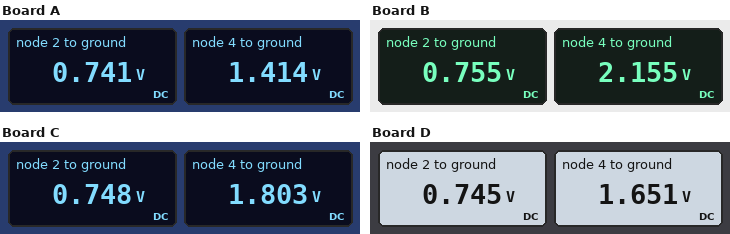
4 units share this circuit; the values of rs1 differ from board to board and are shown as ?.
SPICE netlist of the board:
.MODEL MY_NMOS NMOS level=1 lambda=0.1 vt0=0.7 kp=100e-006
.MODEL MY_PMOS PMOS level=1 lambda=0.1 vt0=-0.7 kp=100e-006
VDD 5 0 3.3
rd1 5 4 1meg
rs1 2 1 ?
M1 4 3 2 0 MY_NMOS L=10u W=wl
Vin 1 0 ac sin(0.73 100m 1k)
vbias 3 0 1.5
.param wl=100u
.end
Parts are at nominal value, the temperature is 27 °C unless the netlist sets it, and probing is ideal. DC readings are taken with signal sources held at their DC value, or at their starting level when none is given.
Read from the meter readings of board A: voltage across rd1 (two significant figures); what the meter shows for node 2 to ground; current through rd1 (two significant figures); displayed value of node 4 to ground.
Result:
1.9 V
0.741 V
1.9 µA
1.414 V
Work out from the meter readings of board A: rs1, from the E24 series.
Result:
5.6 kΩ
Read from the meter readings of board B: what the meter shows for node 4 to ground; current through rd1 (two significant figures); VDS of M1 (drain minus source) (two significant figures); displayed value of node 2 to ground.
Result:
2.155 V
1.1 µA
1.4 V
0.755 V
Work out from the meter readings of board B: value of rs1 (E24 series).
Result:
22 kΩ
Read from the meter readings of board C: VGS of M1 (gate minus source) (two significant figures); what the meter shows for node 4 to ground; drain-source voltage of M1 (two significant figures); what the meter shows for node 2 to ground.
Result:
750 mV
1.803 V
1.1 V
0.748 V
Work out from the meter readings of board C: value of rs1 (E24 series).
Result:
12 kΩ
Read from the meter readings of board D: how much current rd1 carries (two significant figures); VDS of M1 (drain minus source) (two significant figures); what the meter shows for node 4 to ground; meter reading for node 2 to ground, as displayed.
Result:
1.6 µA
910 mV
1.651 V
0.745 V
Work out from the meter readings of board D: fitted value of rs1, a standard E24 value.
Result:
9.1 kΩ
